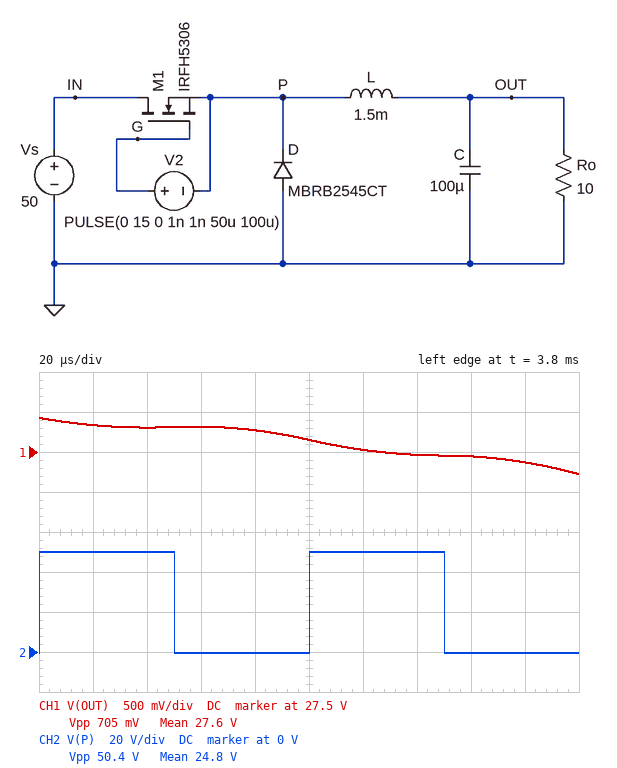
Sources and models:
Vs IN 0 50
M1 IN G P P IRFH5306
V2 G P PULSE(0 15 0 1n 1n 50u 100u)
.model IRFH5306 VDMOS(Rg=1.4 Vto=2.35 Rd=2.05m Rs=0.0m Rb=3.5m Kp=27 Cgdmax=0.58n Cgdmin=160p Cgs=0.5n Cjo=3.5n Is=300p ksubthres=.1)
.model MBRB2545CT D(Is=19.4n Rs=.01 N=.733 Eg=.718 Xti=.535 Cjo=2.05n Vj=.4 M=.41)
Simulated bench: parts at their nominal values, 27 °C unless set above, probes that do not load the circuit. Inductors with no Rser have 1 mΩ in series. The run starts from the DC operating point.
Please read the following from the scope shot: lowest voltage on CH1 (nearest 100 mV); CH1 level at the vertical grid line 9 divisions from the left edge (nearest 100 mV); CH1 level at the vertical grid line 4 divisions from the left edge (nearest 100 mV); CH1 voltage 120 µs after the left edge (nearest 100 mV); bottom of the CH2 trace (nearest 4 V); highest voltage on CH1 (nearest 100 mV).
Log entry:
27.2 V
27.4 V
27.8 V
27.5 V
0 V
27.9 V
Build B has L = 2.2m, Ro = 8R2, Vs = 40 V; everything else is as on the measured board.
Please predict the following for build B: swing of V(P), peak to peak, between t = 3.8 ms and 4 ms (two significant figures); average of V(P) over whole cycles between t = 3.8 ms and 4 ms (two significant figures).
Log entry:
40 V
20 V
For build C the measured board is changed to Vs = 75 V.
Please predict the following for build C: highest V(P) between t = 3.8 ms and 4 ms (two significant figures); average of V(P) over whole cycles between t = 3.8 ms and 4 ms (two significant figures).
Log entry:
75 V
37 V
